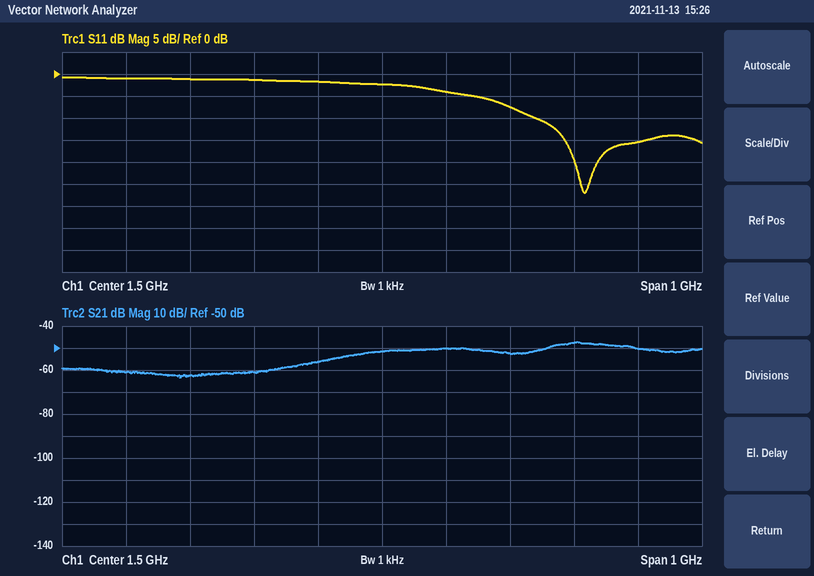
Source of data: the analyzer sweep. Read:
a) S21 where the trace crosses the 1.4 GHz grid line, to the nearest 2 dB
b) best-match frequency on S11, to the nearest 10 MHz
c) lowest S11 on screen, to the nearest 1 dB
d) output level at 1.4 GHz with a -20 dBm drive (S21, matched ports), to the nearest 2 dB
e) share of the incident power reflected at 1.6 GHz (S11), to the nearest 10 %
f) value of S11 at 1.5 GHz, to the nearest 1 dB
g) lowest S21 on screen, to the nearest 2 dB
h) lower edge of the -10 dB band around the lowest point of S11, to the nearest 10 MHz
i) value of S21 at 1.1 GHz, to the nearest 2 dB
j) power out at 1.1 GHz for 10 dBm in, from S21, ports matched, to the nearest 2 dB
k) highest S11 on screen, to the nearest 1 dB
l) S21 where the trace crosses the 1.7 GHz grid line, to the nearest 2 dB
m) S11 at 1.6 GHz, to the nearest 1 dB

-56 dB
1.82 GHz
-27 dB
-76 dBm
40 %
-2 dB
-64 dB
1.74 GHz
-60 dB
-50 dBm
-1 dB
-52 dB
-4 dB
